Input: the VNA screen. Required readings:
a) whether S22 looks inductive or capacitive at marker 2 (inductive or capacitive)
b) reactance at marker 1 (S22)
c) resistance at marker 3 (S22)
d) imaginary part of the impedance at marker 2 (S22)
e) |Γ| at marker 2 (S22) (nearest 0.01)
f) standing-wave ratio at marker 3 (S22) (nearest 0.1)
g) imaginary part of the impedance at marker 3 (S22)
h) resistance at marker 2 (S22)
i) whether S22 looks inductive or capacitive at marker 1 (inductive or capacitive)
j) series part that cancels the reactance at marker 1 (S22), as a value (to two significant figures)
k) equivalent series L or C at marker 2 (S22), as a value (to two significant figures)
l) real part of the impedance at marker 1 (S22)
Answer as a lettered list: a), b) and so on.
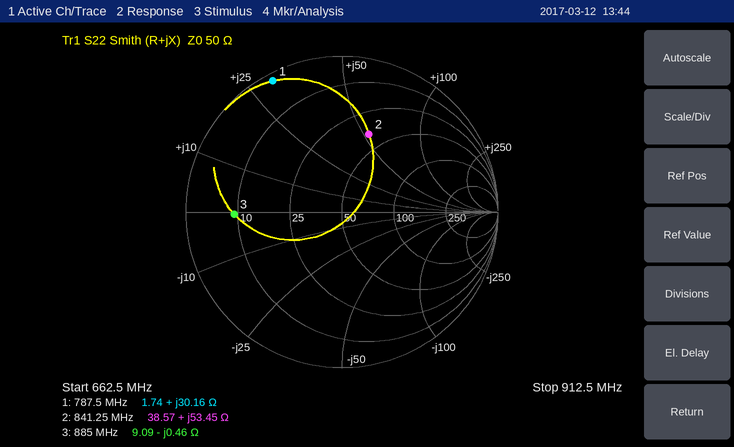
a) inductive
b) +30.16 Ω
c) 9.09 Ω
d) +53.45 Ω
e) 0.53
f) 5.5
g) -0.46 Ω
h) 38.57 Ω
i) inductive
j) 6.7 pF
k) 10 nH
l) 1.74 Ω
